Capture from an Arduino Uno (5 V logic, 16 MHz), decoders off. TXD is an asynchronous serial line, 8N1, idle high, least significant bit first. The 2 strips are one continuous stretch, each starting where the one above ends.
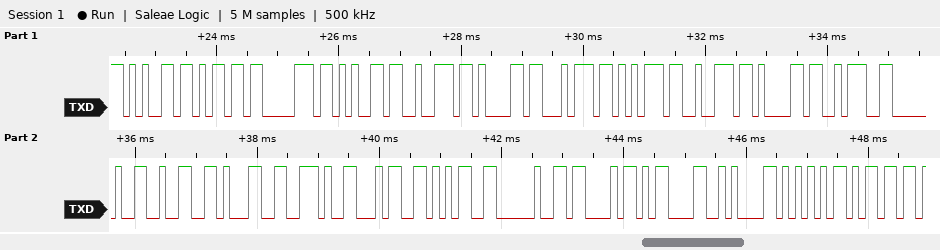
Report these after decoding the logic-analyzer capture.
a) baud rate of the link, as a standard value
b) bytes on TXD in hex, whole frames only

9600 baud
65 6D 70 65 72 61 74 75 72 61 3A 20 32 31 2E 34 35 20 43 0D 0A 55 6D
